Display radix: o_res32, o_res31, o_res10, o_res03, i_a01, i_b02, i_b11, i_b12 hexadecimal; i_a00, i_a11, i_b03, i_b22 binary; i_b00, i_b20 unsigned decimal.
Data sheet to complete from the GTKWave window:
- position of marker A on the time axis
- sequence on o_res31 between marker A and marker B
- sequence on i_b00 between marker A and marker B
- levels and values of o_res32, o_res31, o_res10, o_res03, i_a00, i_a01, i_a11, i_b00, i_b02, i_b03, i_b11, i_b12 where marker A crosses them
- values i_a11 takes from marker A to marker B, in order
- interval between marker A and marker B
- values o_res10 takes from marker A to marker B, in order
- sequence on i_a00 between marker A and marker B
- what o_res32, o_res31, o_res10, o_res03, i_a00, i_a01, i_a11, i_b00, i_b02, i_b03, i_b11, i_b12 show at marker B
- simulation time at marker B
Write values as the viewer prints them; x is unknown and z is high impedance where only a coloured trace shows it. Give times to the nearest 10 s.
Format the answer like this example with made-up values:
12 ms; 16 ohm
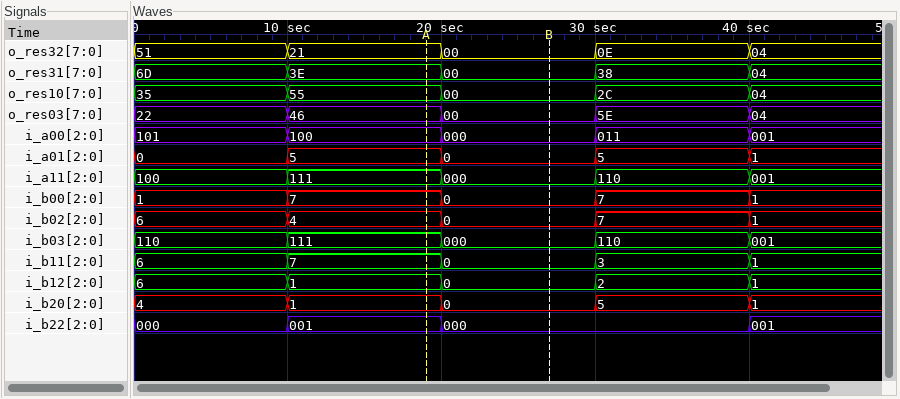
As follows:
20 s; 3E, 00; 7, 0; o_res32=21, o_res31=3E, o_res10=55, o_res03=46, i_a00=100, i_a01=5, i_a11=111, i_b00=7, i_b02=4, i_b03=111, i_b11=7, i_b12=1; 111, 000; 10 s; 55, 00; 100, 000; o_res32=00, o_res31=00, o_res10=00, o_res03=00, i_a00=000, i_a01=0, i_a11=000, i_b00=0, i_b02=0, i_b03=000, i_b11=0, i_b12=0; 30 s
